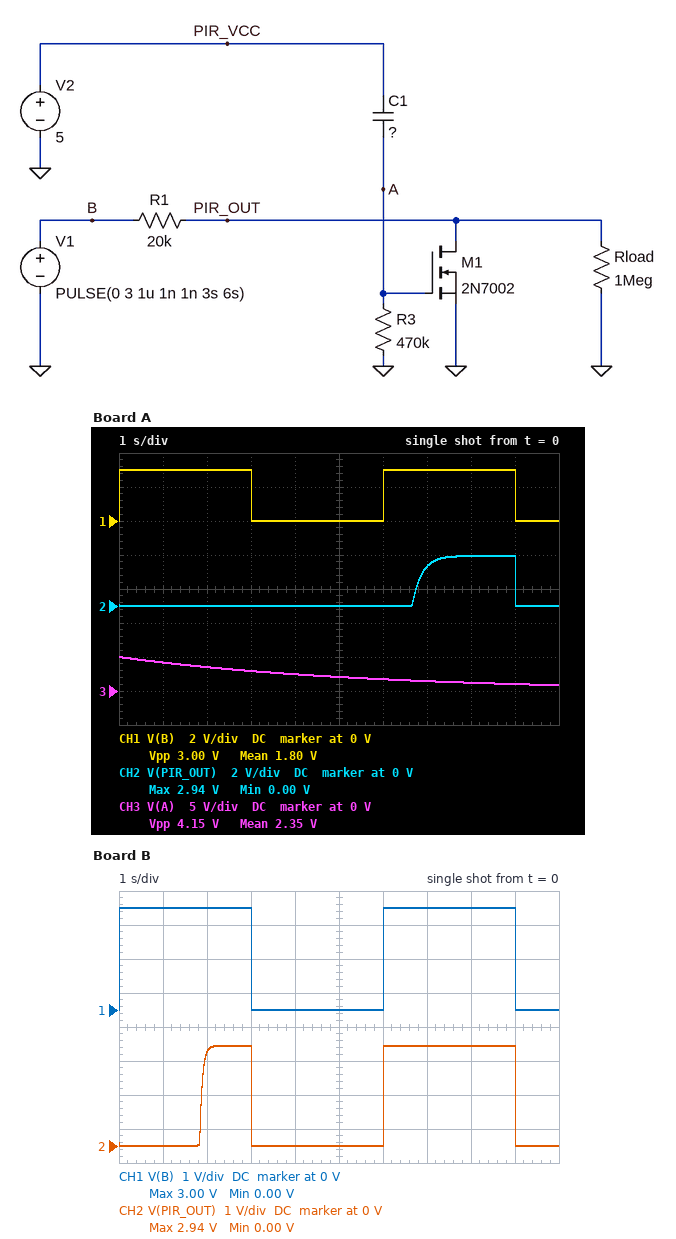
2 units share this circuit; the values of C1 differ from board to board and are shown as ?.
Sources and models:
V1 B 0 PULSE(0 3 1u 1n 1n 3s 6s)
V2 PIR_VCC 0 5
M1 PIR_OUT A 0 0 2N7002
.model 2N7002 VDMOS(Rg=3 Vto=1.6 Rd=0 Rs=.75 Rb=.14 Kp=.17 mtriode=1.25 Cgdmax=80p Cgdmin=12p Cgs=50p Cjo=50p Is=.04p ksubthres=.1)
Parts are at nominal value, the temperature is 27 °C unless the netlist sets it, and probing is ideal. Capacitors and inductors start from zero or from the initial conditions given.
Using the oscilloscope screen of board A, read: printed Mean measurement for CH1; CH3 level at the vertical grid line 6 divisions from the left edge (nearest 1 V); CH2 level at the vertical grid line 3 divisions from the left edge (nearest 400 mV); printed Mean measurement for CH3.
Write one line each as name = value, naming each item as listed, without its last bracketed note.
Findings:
printed Mean measurement for CH1 = 1.80 V
CH3 level at the vertical grid line 6 divisions from the left edge = 2 V
CH2 level at the vertical grid line 3 divisions from the left edge = 0 V
printed Mean measurement for CH3 = 2.35 V
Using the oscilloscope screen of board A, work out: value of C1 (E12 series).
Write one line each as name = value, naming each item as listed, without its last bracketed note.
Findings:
value of C1 = 12 µF
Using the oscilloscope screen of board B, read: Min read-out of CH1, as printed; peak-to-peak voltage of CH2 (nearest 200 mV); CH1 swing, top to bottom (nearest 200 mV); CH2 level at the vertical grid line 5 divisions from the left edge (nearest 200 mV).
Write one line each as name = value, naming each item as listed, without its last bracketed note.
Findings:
Min read-out of CH1, as printed = 0.00 V
peak-to-peak voltage of CH2 = 3.0 V
CH1 swing, top to bottom = 3.0 V
CH2 level at the vertical grid line 5 divisions from the left edge = 0 V
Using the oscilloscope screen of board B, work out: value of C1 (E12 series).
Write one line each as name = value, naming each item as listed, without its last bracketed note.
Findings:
value of C1 = 3.3 µF
